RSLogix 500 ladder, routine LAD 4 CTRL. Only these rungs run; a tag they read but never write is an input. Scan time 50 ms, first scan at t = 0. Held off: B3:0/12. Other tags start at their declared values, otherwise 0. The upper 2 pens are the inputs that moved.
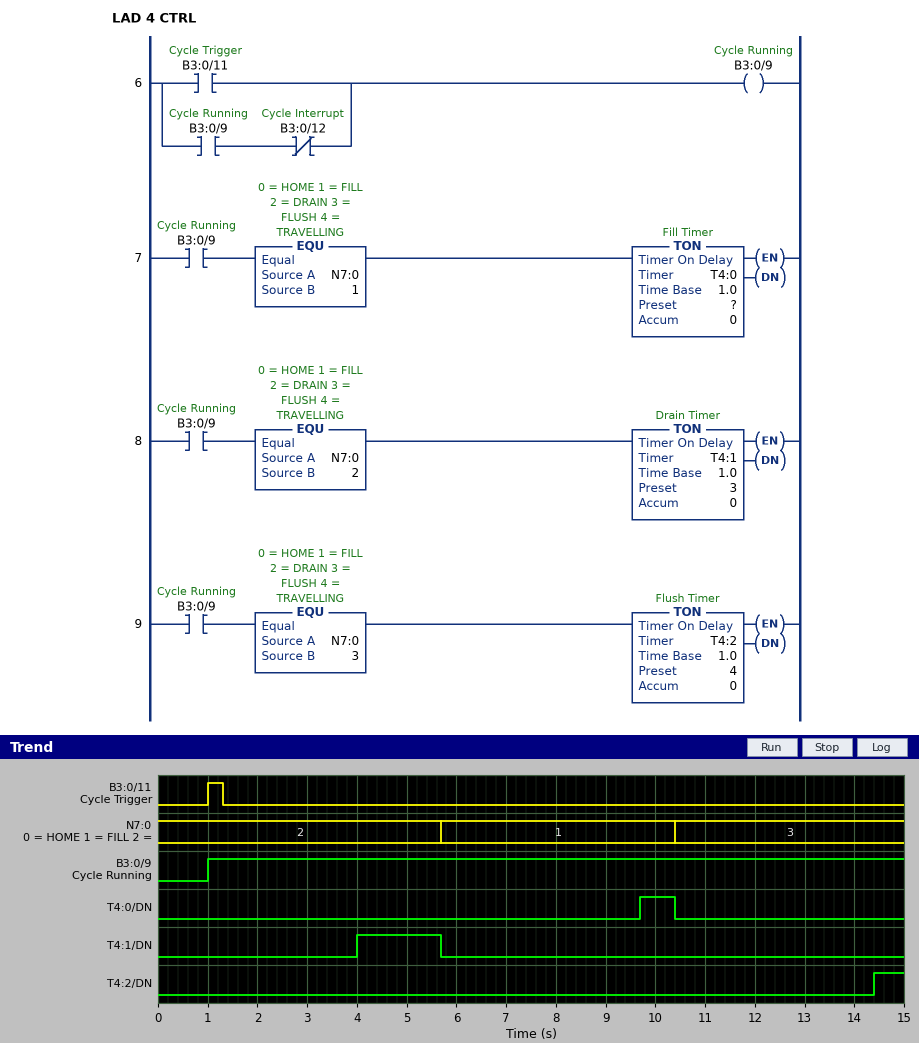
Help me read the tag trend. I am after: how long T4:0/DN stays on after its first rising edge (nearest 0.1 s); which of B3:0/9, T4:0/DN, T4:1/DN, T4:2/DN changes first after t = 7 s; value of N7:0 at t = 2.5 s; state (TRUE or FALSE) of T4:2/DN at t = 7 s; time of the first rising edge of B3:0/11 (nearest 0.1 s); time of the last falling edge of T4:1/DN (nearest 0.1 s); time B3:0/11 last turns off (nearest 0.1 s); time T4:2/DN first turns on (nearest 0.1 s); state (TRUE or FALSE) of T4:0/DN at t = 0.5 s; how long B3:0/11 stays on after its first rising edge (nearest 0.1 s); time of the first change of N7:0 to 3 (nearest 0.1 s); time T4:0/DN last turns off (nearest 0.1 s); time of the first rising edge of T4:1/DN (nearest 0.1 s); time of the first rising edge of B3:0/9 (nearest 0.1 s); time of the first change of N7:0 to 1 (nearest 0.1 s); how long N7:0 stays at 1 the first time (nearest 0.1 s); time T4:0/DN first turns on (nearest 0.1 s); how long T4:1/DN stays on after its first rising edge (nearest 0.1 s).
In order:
0.7 s
T4:0/DN
2
FALSE
1.0 s
5.7 s
1.3 s
14.4 s
FALSE
0.3 s
10.4 s
10.4 s
4.0 s
1.0 s
5.7 s
4.7 s
9.7 s
1.7 s
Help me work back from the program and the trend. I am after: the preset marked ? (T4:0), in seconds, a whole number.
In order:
4 s
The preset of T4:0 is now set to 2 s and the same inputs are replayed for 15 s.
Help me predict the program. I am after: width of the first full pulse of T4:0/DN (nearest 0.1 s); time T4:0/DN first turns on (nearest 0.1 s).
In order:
2.7 s
7.7 s
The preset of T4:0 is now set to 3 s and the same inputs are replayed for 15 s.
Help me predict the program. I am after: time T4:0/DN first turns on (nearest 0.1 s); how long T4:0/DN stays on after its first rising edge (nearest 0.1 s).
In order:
8.7 s
1.7 s
